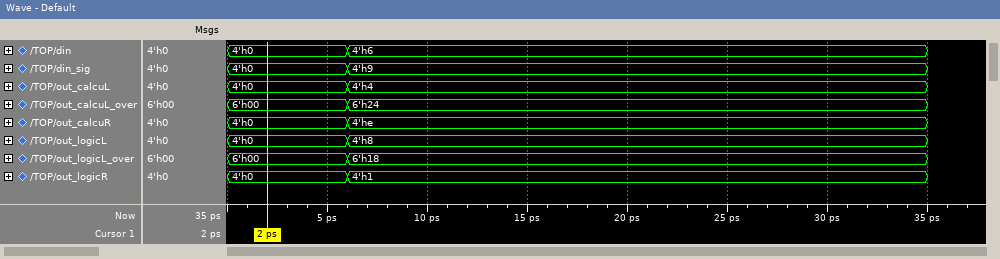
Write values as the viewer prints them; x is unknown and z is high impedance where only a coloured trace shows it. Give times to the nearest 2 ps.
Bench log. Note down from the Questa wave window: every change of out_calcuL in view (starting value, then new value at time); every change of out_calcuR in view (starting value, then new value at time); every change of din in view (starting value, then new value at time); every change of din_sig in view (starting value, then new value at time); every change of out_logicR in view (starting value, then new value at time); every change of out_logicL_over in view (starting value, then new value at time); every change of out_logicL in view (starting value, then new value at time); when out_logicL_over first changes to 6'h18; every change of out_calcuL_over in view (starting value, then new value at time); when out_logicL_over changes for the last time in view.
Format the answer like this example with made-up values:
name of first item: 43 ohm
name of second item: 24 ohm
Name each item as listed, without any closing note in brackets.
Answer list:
every change of out_calcuL in view: 4'h0, 4'h4 at 6 ps
every change of out_calcuR in view: 4'h0, 4'he at 6 ps
every change of din in view: 4'h0, 4'h6 at 6 ps
every change of din_sig in view: 4'h0, 4'h9 at 6 ps
every change of out_logicR in view: 4'h0, 4'h1 at 6 ps
every change of out_logicL_over in view: 6'h00, 6'h18 at 6 ps
every change of out_logicL in view: 4'h0, 4'h8 at 6 ps
when out_logicL_over first changes to 6'h18: 6 ps
every change of out_calcuL_over in view: 6'h00, 6'h24 at 6 ps
when out_logicL_over changes for the last time in view: 6 ps
